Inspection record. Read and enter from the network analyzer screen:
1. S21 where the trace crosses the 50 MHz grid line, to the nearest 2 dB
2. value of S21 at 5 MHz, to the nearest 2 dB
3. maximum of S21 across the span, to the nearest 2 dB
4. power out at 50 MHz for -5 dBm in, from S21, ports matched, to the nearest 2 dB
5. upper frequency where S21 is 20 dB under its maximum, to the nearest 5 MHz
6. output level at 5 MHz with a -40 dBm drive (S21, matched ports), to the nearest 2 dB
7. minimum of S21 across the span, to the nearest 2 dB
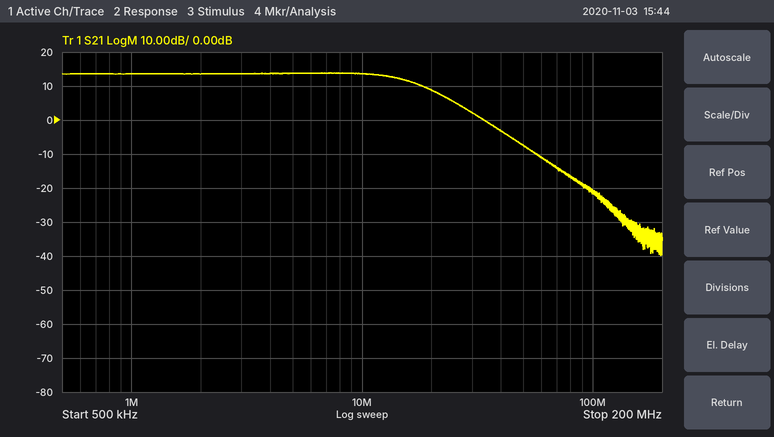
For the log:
-8 dB
14 dB
14 dB
-12 dBm
45 MHz
-26 dBm
-40 dB
